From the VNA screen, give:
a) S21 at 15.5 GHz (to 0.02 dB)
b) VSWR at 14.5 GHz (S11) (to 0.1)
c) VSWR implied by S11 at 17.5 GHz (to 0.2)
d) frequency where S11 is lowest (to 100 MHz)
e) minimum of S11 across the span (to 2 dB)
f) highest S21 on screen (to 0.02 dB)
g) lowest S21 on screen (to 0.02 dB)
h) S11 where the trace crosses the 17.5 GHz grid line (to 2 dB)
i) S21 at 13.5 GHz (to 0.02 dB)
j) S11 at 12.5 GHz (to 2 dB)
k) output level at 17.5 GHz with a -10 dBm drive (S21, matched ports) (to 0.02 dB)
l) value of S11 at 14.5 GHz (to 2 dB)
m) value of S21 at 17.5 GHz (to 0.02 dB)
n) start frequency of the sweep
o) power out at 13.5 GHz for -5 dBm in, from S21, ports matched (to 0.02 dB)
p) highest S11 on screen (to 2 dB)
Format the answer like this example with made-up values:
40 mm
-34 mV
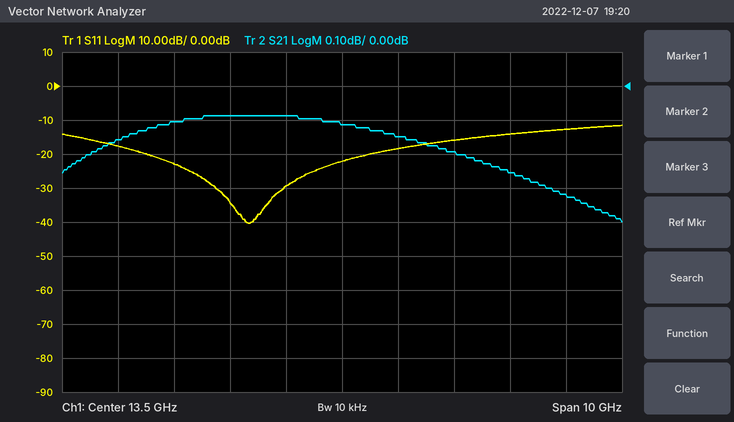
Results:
-0.20 dB
1.3
1.6
11.8 GHz
-40 dB
-0.08 dB
-0.40 dB
-12 dB
-0.12 dB
-30 dB
-10.32 dBm
-18 dB
-0.32 dB
8.5 GHz
-5.12 dBm
-12 dB
